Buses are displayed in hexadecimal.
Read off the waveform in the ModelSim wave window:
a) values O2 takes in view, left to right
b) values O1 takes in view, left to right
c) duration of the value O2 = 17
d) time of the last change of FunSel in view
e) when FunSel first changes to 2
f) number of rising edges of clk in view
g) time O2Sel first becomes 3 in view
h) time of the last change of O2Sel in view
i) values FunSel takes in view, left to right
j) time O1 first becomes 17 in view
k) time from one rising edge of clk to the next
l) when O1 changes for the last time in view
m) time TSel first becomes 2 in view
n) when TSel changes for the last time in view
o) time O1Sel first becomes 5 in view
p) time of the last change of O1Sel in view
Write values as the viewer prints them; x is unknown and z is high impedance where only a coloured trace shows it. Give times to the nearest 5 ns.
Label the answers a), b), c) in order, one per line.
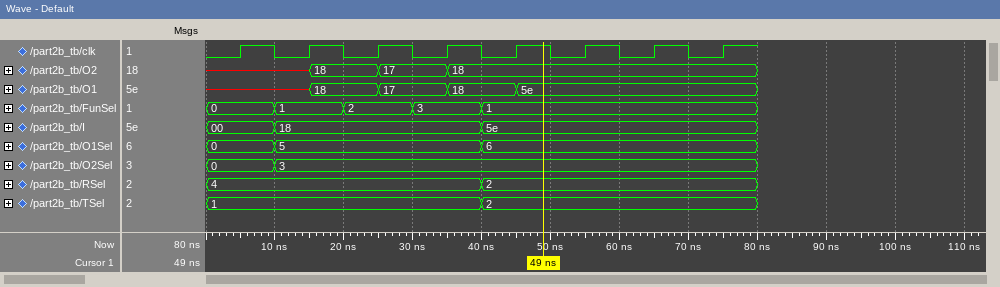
a) x, 18, 17, 18
b) x, 18, 17, 18, 5e
c) 10 ns
d) 40 ns
e) 20 ns
f) 8
g) 10 ns
h) 10 ns
i) 0, 1, 2, 3, 1
j) 25 ns
k) 10 ns
l) 45 ns
m) 40 ns
n) 40 ns
o) 10 ns
p) 40 ns
